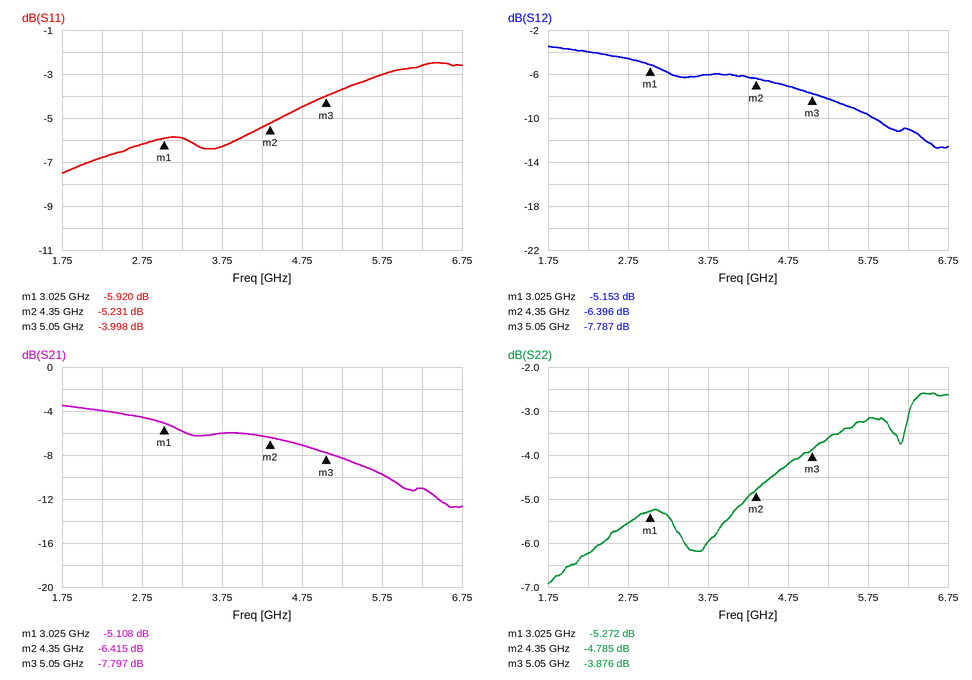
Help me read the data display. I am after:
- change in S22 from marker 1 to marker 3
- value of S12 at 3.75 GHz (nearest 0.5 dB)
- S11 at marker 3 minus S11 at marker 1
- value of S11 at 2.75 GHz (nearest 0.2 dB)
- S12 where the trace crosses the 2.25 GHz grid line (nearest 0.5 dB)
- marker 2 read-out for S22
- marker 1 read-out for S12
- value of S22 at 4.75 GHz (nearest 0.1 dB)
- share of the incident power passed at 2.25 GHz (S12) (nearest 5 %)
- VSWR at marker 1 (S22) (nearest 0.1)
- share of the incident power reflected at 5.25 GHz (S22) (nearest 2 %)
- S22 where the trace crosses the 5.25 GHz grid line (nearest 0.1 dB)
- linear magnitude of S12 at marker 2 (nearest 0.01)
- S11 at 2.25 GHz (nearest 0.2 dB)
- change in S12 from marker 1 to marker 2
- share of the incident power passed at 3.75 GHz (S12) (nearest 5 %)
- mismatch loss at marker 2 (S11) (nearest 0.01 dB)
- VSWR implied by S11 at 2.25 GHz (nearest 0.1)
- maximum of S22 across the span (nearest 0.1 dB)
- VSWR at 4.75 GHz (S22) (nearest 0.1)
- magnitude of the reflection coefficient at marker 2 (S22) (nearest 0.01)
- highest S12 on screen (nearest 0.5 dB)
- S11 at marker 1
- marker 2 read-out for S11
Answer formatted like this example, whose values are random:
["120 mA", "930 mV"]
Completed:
["1.396 dB", "-6.0 dB", "1.922 dB", "-6.2 dB", "-4.0 dB", "-4.785 dB", "-5.153 dB", "-4.2 dB", "40 %", "3.4", "44 %", "-3.6 dB", "0.48", "-6.8 dB", "-1.243 dB", "25 %", "1.55 dB", "2.7", "-2.6 dB", "4.2", "0.58", "-3.5 dB", "-5.920 dB", "-5.231 dB"]
